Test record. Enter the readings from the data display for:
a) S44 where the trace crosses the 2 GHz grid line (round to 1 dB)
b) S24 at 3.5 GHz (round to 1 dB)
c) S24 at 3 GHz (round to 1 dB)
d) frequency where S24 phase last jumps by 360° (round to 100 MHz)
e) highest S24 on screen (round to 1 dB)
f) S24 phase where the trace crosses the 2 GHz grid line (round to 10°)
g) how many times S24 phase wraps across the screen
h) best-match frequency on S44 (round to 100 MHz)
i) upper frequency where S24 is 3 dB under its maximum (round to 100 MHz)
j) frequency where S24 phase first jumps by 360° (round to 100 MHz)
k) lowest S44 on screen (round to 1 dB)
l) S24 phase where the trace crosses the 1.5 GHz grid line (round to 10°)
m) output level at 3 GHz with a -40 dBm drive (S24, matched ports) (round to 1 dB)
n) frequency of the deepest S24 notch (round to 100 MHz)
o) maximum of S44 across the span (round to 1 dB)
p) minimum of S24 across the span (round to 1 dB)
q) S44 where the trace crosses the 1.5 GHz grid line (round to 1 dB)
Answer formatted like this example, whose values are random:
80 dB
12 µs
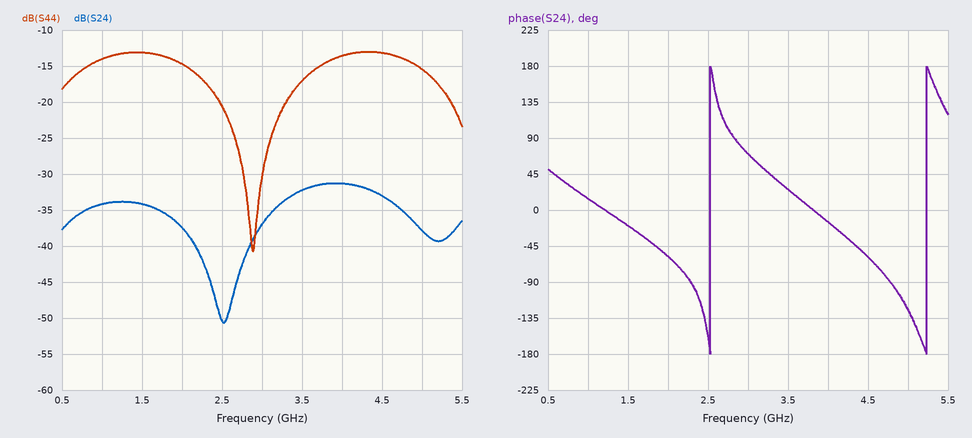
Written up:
-15 dB
-32 dB
-37 dB
5.2 GHz
-31 dB
-60°
2
2.9 GHz
4.7 GHz
2.5 GHz
-41 dB
-20°
-77 dBm
2.5 GHz
-13 dB
-51 dB
-13 dB
